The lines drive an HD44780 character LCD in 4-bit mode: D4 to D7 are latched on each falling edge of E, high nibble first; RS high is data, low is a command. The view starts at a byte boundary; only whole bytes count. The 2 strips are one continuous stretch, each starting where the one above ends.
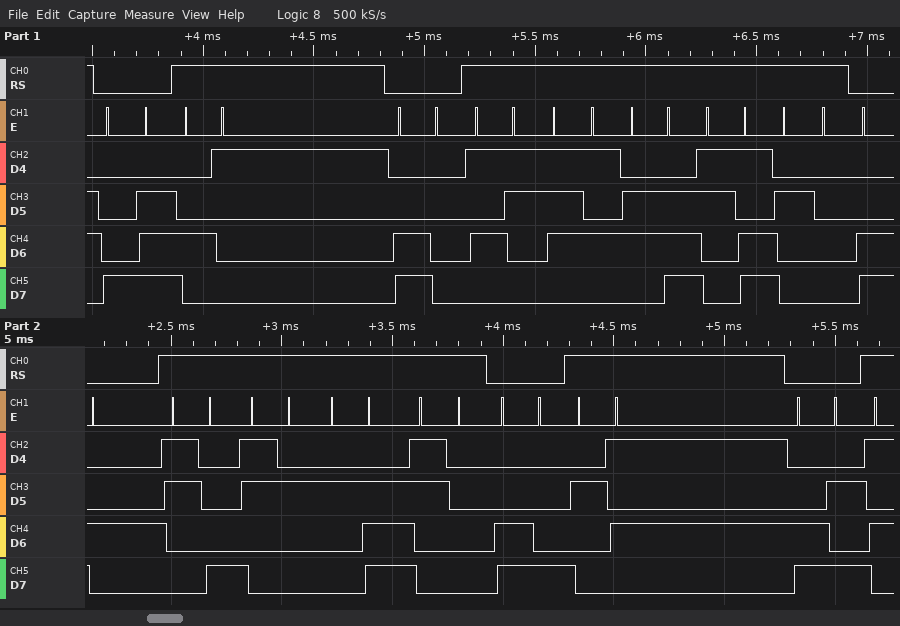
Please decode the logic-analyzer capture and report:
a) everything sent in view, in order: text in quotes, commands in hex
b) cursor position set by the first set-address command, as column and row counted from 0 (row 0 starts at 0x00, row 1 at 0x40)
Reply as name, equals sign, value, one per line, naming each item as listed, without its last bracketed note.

everything sent in view, in order: text in quotes, commands in hex = 0x8E "A" 0xC0 "Sun= " 0xC4 "82.0" 0xC8 "%" 0xCA
cursor position set by the first set-address command, as column and row counted from 0 = column 14, row 0
